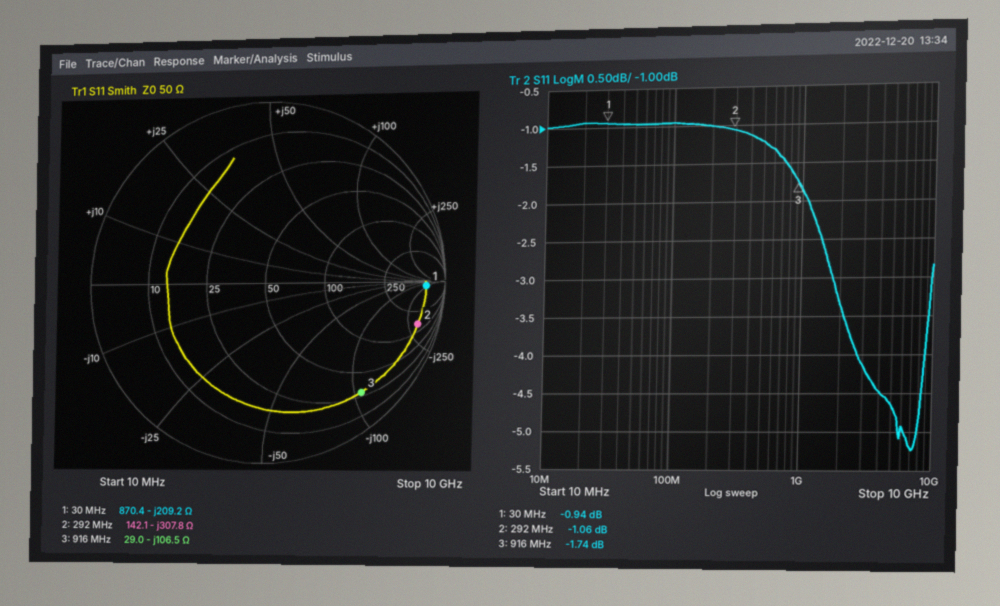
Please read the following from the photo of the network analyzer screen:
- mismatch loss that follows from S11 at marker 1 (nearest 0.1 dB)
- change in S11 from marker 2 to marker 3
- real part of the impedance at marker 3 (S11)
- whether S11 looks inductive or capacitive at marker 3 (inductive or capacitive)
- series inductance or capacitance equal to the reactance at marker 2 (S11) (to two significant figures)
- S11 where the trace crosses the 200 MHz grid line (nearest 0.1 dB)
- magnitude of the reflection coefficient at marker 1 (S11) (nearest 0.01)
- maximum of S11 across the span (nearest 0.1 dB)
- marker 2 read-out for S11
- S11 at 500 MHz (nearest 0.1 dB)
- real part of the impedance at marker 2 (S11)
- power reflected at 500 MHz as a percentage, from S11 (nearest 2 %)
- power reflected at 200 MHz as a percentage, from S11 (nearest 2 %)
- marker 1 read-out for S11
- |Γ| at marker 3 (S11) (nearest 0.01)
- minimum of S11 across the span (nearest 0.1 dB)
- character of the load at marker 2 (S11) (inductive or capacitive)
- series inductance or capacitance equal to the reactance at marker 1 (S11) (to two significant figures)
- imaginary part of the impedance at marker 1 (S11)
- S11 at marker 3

7.1 dB
-0.68 dB
29.0 Ω
capacitive
1.8 pF
-1.0 dB
0.90
-0.9 dB
-1.06 dB
-1.2 dB
142.1 Ω
76 %
80 %
-0.94 dB
0.82
-5.2 dB
capacitive
25 pF
-209.2 Ω
-1.74 dB
